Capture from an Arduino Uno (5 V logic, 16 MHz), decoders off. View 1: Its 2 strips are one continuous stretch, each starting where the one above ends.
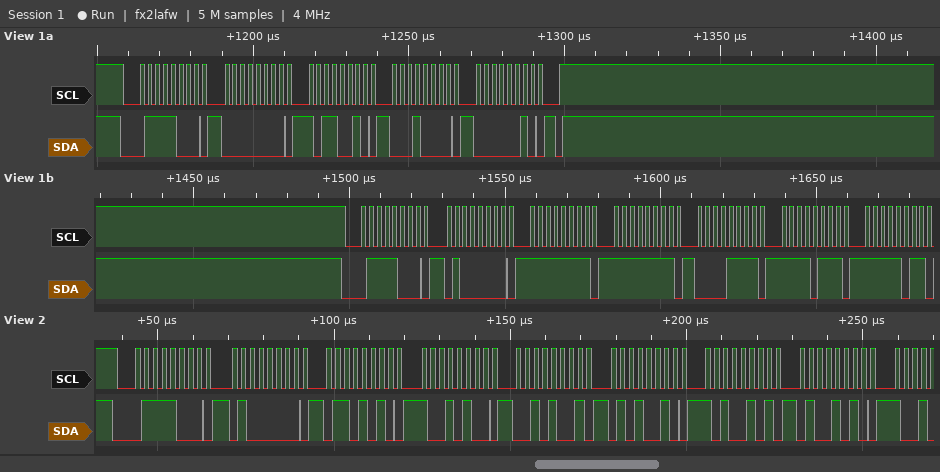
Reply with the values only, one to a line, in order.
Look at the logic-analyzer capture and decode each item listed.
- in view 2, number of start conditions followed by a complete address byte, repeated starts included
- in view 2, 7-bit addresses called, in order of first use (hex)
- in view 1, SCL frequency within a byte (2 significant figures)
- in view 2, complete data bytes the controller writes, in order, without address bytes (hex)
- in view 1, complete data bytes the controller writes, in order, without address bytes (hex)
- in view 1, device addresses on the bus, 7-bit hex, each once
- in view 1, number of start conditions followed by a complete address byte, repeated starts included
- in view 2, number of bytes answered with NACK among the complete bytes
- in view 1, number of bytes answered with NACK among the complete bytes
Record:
1
0x3C
400 kHz
40 6A 94 29 52 A5 4A
00 B2 10 02 40 FF FF 0F F7 FB
0x3C
2
0
0
